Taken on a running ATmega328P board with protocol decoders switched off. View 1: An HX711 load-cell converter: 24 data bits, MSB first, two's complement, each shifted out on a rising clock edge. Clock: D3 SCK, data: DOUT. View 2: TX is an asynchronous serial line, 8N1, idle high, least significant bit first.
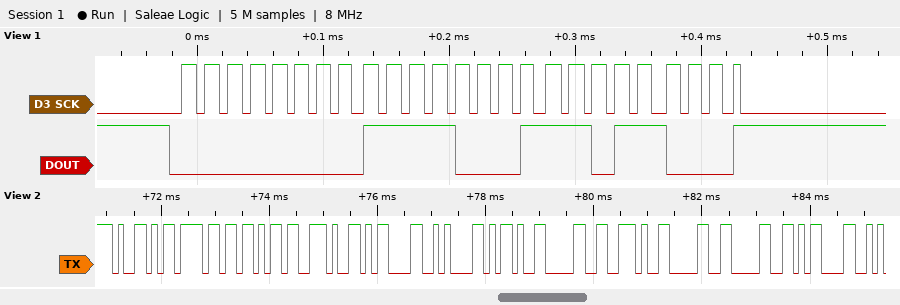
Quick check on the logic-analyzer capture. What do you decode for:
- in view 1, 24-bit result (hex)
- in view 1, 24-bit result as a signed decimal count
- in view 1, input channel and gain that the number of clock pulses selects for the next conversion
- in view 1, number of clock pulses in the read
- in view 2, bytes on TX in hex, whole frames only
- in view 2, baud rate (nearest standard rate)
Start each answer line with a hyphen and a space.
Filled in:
- 0x00F1D8
- 61912
- channel A, gain 128
- 25
- 59 6F 6B 2E 0D 0A 2D 30 2E 30 30 0D
- 9600 baud
